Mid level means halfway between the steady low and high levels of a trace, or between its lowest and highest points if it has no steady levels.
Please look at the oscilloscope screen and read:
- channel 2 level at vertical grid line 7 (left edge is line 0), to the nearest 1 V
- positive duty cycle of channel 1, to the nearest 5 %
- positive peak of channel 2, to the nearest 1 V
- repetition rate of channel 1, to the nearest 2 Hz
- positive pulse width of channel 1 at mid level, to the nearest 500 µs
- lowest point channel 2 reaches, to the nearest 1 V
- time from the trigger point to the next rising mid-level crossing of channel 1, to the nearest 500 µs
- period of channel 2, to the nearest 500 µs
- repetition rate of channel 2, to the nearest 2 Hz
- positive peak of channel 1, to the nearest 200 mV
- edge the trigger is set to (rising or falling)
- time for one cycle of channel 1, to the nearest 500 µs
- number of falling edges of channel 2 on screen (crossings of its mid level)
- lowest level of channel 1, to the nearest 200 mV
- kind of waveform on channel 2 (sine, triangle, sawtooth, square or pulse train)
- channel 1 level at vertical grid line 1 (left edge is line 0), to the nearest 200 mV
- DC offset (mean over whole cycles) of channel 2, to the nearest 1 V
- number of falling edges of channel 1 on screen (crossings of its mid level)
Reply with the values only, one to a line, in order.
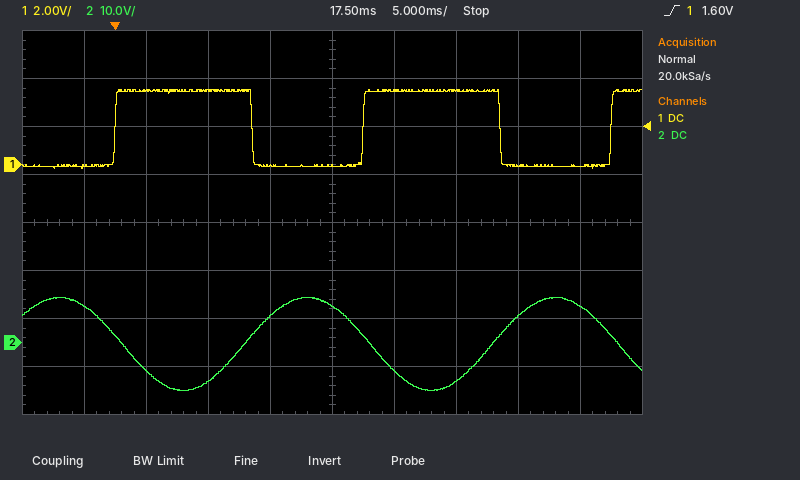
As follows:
-8 V
55 %
9 V
50 Hz
11.0 ms
-10 V
20.0 ms
20.0 ms
50 Hz
3.2 V
rising
20.0 ms
3
-200 mV
sine
0.0 V
0 V
2
